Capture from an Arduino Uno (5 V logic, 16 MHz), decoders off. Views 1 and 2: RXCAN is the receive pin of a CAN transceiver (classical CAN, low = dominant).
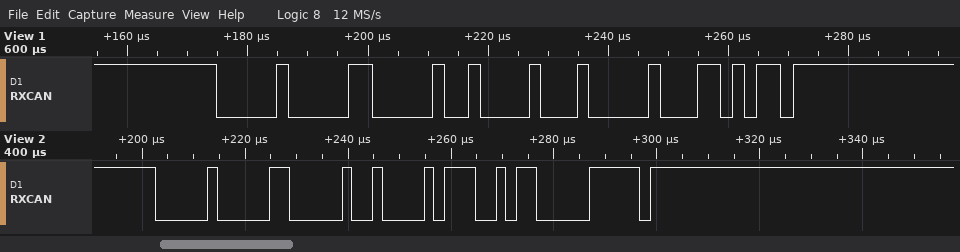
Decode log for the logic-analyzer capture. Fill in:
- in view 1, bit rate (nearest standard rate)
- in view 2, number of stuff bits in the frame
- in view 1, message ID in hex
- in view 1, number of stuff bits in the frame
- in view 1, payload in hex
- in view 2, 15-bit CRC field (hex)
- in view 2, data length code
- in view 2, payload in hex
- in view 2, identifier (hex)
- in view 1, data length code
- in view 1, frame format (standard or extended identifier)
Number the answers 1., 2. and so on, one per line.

1. 500 kbit/s
2. 4
3. 0x002
4. 4
5. 08
6. 0x4B07
7. 1
8. 0B
9. 0x002
10. 1
11. standard
